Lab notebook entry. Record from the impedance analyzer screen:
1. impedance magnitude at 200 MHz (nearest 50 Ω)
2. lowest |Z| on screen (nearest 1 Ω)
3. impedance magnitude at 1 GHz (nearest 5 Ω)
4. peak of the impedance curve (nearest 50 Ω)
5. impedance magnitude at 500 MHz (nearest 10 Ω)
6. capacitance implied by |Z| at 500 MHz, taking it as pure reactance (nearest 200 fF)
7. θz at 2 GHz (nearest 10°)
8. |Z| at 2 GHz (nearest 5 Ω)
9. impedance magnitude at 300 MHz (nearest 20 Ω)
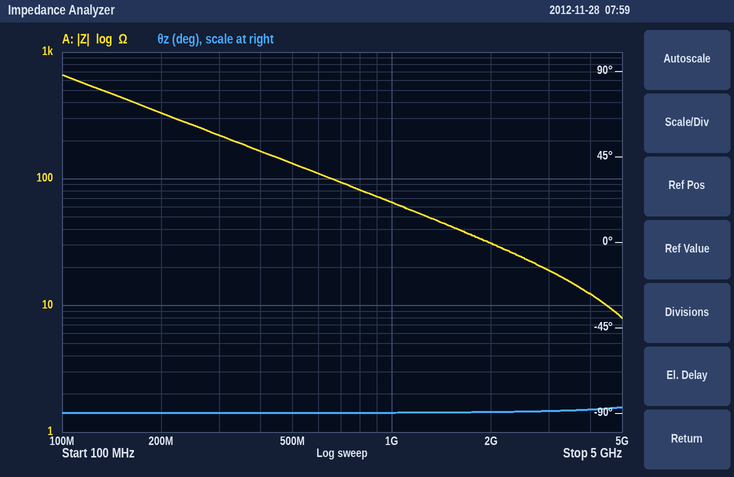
350 Ω
8 Ω
65 Ω
650 Ω
130 Ω
2.4 pF
-90°
30 Ω
220 Ω
